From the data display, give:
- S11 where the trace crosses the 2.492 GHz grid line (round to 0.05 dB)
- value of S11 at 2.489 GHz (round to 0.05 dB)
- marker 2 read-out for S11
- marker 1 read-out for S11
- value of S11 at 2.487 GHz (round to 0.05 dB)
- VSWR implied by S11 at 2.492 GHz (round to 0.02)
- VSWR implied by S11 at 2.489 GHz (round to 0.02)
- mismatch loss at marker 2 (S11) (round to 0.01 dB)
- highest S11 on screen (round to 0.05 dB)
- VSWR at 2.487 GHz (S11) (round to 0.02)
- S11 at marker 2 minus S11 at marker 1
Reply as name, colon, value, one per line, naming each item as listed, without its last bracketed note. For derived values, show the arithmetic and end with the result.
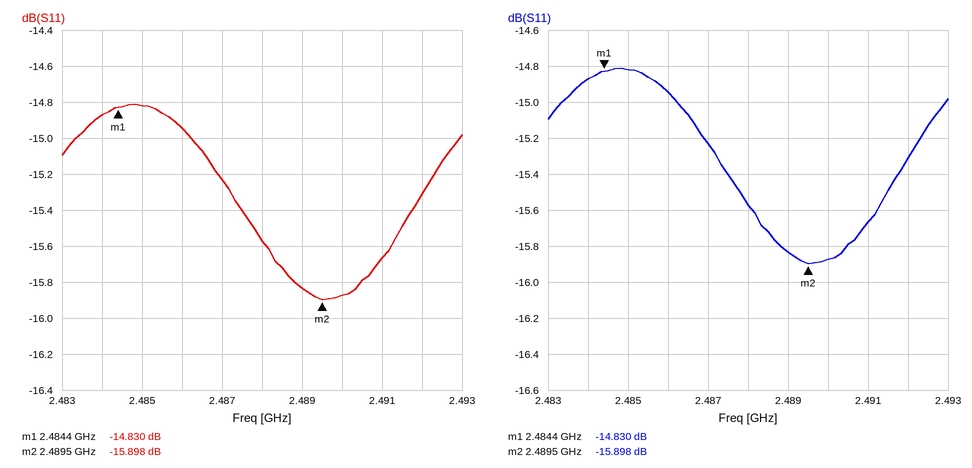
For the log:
S11 where the trace crosses the 2.492 GHz grid line: -15.30 dB
value of S11 at 2.489 GHz: -15.85 dB
marker 2 read-out for S11: -15.898 dB
marker 1 read-out for S11: -14.830 dB
value of S11 at 2.487 GHz: -15.25 dB
VSWR implied by S11 at 2.492 GHz: |Γ| = 10^(-15.3/20) = 0.1718; VSWR = (1 + 0.1718)/(1 − 0.1718) ≈ 1.41, so 1.42 to the nearest 0.02
VSWR implied by S11 at 2.489 GHz: |Γ| = 10^(-15.85/20) = 0.1613; VSWR = (1 + 0.1613)/(1 − 0.1613) ≈ 1.38
mismatch loss at marker 2 (S11): −10 log10(1 − 10^(-15.898/10)) ≈ 0.11 dB
highest S11 on screen: -14.80 dB
VSWR at 2.487 GHz (S11): |Γ| = 10^(-15.25/20) = 0.1728; VSWR = (1 + 0.1728)/(1 − 0.1728) ≈ 1.42
S11 at marker 2 minus S11 at marker 1: -15.898 − (-14.83) = -1.068 dB
